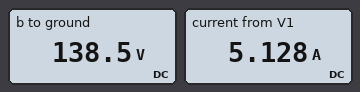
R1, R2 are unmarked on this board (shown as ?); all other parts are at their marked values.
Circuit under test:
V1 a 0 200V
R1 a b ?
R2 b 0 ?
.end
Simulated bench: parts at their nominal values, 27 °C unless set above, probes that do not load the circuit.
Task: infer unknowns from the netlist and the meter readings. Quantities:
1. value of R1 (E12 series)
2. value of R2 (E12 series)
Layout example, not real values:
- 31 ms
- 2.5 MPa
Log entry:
- 12 Ω
- 27 Ω
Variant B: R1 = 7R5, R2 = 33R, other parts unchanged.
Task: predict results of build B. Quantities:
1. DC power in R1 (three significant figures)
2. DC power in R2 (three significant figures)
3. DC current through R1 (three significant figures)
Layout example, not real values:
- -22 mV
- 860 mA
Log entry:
- 183 W
- 805 W
- 4.94 A
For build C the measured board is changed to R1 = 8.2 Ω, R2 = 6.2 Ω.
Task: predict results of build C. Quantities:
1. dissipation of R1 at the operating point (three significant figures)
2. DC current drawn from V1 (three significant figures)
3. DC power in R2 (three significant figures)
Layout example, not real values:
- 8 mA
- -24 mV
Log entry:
- 1.58 kW
- 13.9 A
- 1.20 kW
